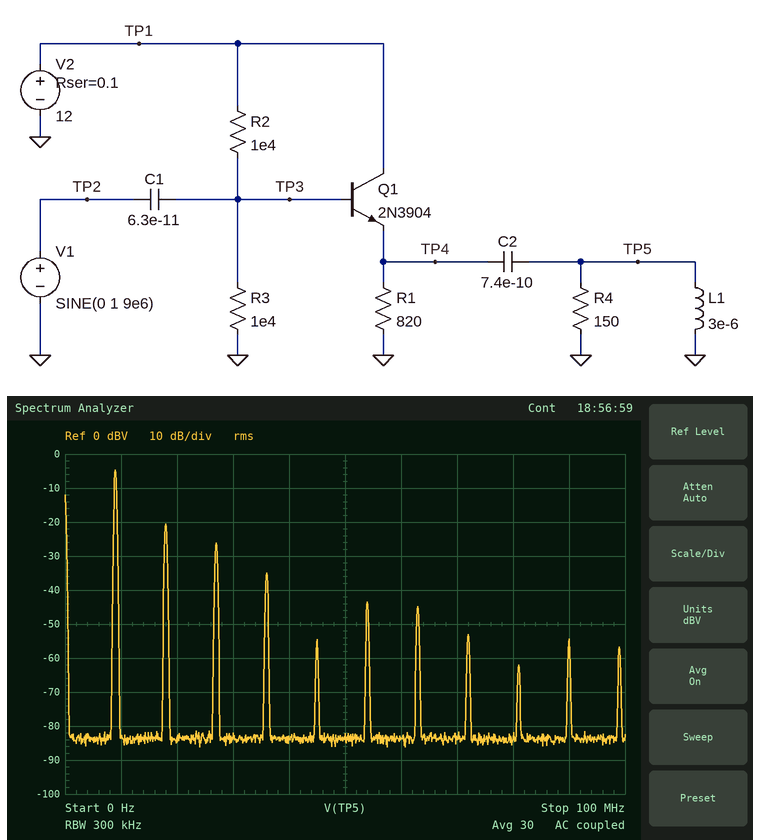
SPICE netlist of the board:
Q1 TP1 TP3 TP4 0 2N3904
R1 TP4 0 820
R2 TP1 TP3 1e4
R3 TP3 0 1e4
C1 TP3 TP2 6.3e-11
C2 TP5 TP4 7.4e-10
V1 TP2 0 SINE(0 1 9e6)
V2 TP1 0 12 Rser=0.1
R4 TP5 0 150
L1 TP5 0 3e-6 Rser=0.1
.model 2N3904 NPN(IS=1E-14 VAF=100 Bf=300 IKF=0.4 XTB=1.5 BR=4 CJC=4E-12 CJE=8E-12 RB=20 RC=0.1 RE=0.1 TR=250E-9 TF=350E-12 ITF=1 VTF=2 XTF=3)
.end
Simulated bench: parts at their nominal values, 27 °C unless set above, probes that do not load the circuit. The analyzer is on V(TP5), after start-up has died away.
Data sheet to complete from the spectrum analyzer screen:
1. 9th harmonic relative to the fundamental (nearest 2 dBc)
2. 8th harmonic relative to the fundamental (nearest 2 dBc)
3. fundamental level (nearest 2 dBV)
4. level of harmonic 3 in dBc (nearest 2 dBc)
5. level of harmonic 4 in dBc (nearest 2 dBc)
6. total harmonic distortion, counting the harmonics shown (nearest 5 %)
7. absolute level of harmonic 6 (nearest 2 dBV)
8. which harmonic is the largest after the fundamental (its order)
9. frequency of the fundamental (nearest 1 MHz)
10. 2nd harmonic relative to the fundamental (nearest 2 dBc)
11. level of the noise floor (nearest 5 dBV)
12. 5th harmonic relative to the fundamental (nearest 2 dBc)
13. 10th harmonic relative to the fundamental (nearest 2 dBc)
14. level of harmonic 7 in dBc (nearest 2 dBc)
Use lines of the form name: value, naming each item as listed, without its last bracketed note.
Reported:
9th harmonic relative to the fundamental: -58 dBc
8th harmonic relative to the fundamental: -48 dBc
fundamental level: -4 dBV
level of harmonic 3 in dBc: -22 dBc
level of harmonic 4 in dBc: -30 dBc
total harmonic distortion, counting the harmonics shown: 20 %
absolute level of harmonic 6: -44 dBV
which harmonic is the largest after the fundamental: 2
frequency of the fundamental: 9 MHz
2nd harmonic relative to the fundamental: -16 dBc
level of the noise floor: -85 dBV
5th harmonic relative to the fundamental: -50 dBc
10th harmonic relative to the fundamental: -50 dBc
level of harmonic 7 in dBc: -40 dBc
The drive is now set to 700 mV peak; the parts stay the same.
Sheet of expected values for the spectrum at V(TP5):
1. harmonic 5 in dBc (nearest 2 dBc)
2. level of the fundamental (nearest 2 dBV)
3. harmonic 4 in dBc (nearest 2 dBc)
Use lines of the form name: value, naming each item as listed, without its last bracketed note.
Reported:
harmonic 5 in dBc: -46 dBc
level of the fundamental: -6 dBV
harmonic 4 in dBc: -40 dBc
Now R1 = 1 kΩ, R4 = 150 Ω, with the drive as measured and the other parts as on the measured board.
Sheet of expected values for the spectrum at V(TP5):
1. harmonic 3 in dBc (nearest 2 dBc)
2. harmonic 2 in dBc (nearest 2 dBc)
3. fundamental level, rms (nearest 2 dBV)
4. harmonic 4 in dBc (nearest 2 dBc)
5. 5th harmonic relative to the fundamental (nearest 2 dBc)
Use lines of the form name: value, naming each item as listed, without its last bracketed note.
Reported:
harmonic 3 in dBc: -20 dBc
harmonic 2 in dBc: -12 dBc
fundamental level, rms: -6 dBV
harmonic 4 in dBc: -36 dBc
5th harmonic relative to the fundamental: -34 dBc
